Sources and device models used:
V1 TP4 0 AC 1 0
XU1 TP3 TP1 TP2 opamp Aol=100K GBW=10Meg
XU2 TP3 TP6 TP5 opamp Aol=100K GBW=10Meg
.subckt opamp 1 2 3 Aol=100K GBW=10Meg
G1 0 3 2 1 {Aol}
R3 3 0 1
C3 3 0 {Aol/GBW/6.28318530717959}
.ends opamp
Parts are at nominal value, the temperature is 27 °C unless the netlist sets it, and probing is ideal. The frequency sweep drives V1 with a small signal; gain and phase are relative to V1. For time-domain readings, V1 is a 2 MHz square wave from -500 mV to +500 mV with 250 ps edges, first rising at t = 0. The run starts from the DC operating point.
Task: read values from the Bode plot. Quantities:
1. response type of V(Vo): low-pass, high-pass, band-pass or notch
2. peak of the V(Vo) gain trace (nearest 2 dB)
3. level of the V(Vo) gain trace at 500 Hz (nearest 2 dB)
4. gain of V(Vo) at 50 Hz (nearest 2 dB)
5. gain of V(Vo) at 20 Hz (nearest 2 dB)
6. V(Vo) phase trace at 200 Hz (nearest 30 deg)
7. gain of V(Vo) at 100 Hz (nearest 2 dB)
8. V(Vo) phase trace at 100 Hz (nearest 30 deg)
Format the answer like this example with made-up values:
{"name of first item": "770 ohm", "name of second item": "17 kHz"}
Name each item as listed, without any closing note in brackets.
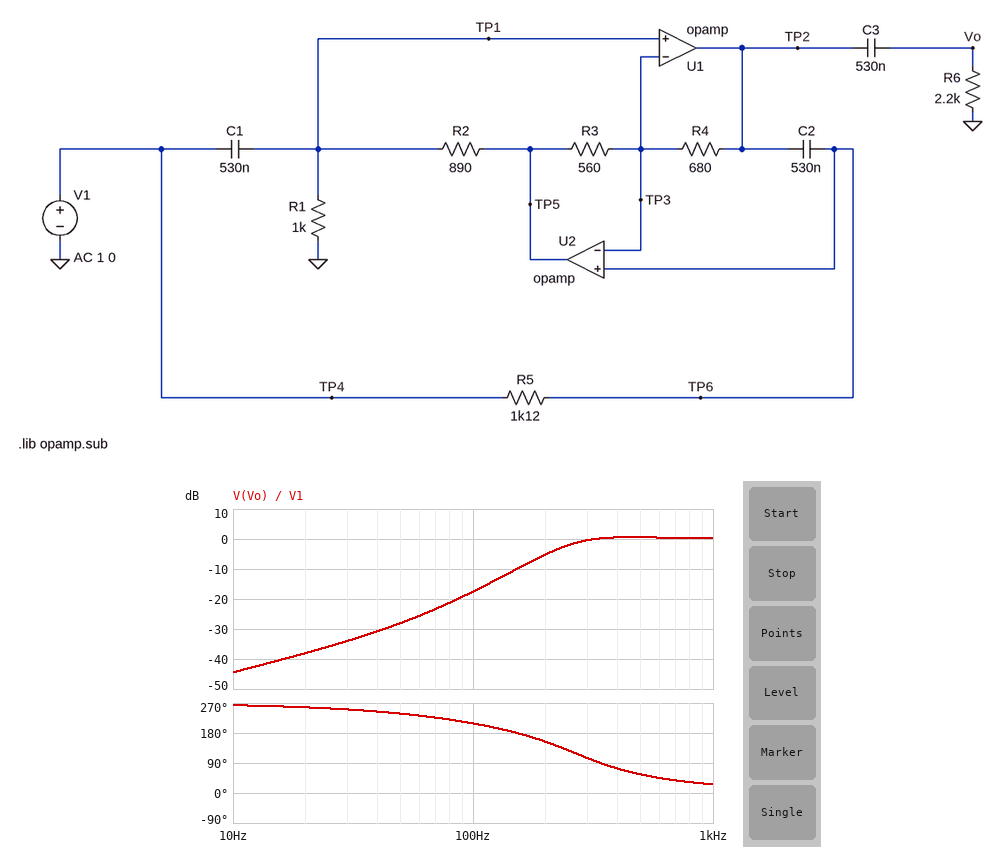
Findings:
{"response type of V(Vo): low-pass, high-pass, band-pass or notch": "high-pass", "peak of the V(Vo) gain trace": "0 dB", "level of the V(Vo) gain trace at 500 Hz": "0 dB", "gain of V(Vo) at 50 Hz": "-28 dB", "gain of V(Vo) at 20 Hz": "-38 dB", "V(Vo) phase trace at 200 Hz": "150 deg", "gain of V(Vo) at 100 Hz": "-18 dB", "V(Vo) phase trace at 100 Hz": "210 deg"}
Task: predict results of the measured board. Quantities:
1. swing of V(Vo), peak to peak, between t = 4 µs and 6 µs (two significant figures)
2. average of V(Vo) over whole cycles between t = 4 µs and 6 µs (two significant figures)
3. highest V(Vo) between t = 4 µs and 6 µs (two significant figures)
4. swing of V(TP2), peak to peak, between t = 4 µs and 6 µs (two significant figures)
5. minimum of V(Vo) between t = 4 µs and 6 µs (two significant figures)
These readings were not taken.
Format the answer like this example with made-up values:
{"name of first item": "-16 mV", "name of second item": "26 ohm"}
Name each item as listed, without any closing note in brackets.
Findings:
{"swing of V(Vo), peak to peak, between t = 4 µs and 6 µs": "1.4 V", "average of V(Vo) over whole cycles between t = 4 µs and 6 µs": "490 mV", "highest V(Vo) between t = 4 µs and 6 µs": "1.2 V", "swing of V(TP2), peak to peak, between t = 4 µs and 6 µs": "1.4 V", "minimum of V(Vo) between t = 4 µs and 6 µs": "-230 mV"}
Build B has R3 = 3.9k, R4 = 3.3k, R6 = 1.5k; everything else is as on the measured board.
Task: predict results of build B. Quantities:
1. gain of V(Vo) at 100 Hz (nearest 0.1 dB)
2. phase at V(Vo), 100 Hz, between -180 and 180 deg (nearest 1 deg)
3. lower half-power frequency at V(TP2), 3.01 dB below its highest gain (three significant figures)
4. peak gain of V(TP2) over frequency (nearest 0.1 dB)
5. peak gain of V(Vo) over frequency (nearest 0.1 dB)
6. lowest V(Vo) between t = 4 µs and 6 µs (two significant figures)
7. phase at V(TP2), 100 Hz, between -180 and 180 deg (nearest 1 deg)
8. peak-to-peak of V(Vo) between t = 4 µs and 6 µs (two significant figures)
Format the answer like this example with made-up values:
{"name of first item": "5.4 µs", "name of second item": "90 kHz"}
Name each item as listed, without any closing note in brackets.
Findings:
{"gain of V(Vo) at 100 Hz": "-22.8 dB", "phase at V(Vo), 100 Hz, between -180 and 180 deg": "46 deg", "lower half-power frequency at V(TP2), 3.01 dB below its highest gain": "314 Hz", "peak gain of V(TP2) over frequency": "0.7 dB", "peak gain of V(Vo) over frequency": "0.2 dB", "lowest V(Vo) between t = 4 µs and 6 µs": "-210 mV", "phase at V(TP2), 100 Hz, between -180 and 180 deg": "-17 deg", "peak-to-peak of V(Vo) between t = 4 µs and 6 µs": "1.4 V"}
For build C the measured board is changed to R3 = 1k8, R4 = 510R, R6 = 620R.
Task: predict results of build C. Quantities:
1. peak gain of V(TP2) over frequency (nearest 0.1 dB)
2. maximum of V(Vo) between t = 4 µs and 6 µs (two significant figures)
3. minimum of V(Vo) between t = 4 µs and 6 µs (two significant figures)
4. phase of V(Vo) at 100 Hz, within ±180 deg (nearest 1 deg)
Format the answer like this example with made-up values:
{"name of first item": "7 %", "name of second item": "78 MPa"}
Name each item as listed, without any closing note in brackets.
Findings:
{"peak gain of V(TP2) over frequency": "0.2 dB", "maximum of V(Vo) between t = 4 µs and 6 µs": "1.1 V", "minimum of V(Vo) between t = 4 µs and 6 µs": "-140 mV", "phase of V(Vo) at 100 Hz, within ±180 deg": "73 deg"}
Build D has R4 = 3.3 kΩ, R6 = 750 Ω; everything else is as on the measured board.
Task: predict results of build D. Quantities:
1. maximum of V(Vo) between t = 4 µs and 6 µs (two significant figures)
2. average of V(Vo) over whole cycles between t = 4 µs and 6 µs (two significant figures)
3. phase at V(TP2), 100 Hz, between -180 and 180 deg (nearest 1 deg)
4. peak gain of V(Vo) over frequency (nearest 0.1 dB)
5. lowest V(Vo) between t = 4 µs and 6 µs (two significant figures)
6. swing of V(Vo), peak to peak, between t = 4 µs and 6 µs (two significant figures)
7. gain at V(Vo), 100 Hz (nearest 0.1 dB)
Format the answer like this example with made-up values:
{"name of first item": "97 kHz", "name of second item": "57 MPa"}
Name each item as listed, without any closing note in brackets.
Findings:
{"maximum of V(Vo) between t = 4 µs and 6 µs": "1.3 V", "average of V(Vo) over whole cycles between t = 4 µs and 6 µs": "490 mV", "phase at V(TP2), 100 Hz, between -180 and 180 deg": "100 deg", "peak gain of V(Vo) over frequency": "0 dB", "lowest V(Vo) between t = 4 µs and 6 µs": "-290 mV", "swing of V(Vo), peak to peak, between t = 4 µs and 6 µs": "1.6 V", "gain at V(Vo), 100 Hz": "-4.5 dB"}
